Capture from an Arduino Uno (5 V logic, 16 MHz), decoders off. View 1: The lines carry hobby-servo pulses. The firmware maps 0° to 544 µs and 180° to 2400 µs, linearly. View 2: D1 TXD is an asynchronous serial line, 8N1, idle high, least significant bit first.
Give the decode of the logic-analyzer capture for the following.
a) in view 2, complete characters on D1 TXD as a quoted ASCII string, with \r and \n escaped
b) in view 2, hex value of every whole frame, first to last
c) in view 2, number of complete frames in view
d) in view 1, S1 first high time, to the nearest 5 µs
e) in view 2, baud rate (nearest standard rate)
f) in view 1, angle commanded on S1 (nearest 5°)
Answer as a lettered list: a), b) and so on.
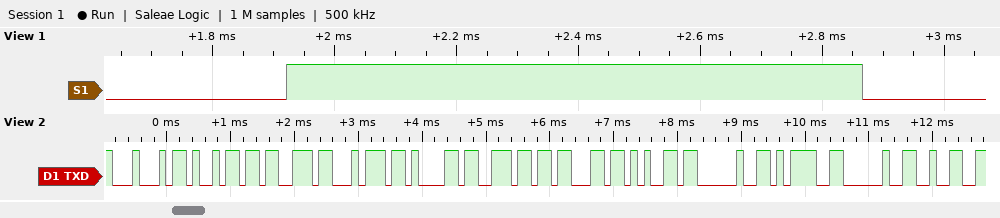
a) "Distance = 2"
b) 0x44 0x69 0x73 0x74 0x61 0x6E 0x63 0x65 0x20 0x3D 0x20 0x32
c) 12
d) 945 µs
e) 9600 baud
f) 40°
